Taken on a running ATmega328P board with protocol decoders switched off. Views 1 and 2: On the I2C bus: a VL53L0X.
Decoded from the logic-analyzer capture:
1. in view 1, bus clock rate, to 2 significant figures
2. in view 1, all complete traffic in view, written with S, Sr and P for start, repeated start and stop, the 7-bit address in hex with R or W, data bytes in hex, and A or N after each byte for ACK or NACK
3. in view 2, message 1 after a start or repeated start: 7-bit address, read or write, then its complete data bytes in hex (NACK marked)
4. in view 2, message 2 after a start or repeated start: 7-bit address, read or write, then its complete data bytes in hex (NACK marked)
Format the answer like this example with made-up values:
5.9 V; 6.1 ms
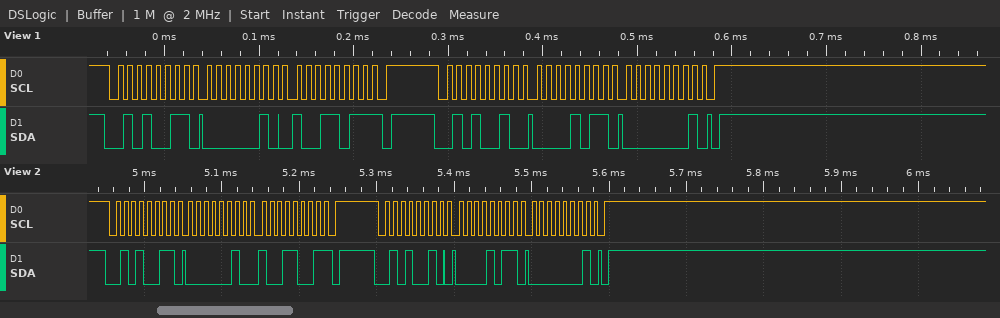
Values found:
100 kHz; S 29R A 02 A 9B N P S 29W A 0B A 01 A P; 0x29 read: 02 99 NACK; 0x29 write: 0B 01
